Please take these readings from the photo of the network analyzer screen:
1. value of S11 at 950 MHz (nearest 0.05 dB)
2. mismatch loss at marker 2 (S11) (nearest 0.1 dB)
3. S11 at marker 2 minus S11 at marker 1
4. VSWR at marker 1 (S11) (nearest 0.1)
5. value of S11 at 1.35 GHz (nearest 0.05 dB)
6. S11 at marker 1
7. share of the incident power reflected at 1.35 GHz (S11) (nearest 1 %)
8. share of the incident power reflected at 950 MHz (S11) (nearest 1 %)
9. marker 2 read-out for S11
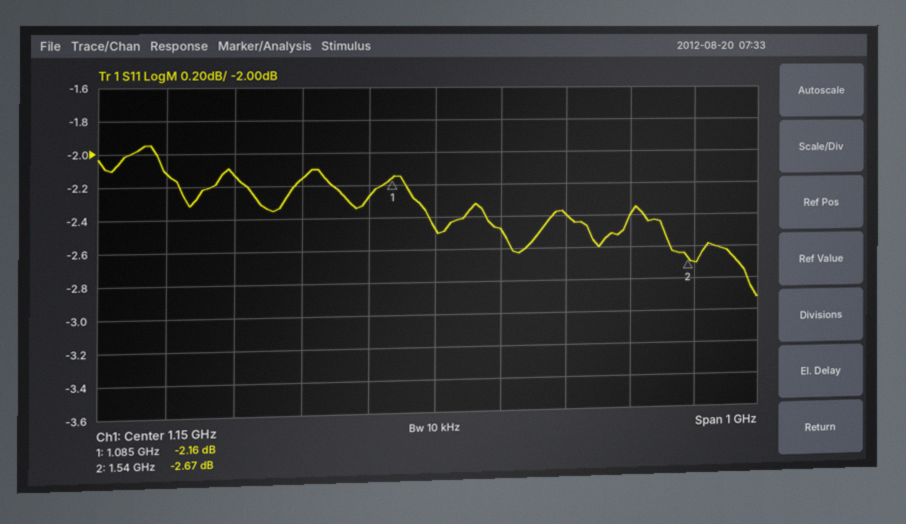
-2.15 dB
3.4 dB
-0.51 dB
8.1
-2.40 dB
-2.16 dB
58 %
61 %
-2.67 dB
